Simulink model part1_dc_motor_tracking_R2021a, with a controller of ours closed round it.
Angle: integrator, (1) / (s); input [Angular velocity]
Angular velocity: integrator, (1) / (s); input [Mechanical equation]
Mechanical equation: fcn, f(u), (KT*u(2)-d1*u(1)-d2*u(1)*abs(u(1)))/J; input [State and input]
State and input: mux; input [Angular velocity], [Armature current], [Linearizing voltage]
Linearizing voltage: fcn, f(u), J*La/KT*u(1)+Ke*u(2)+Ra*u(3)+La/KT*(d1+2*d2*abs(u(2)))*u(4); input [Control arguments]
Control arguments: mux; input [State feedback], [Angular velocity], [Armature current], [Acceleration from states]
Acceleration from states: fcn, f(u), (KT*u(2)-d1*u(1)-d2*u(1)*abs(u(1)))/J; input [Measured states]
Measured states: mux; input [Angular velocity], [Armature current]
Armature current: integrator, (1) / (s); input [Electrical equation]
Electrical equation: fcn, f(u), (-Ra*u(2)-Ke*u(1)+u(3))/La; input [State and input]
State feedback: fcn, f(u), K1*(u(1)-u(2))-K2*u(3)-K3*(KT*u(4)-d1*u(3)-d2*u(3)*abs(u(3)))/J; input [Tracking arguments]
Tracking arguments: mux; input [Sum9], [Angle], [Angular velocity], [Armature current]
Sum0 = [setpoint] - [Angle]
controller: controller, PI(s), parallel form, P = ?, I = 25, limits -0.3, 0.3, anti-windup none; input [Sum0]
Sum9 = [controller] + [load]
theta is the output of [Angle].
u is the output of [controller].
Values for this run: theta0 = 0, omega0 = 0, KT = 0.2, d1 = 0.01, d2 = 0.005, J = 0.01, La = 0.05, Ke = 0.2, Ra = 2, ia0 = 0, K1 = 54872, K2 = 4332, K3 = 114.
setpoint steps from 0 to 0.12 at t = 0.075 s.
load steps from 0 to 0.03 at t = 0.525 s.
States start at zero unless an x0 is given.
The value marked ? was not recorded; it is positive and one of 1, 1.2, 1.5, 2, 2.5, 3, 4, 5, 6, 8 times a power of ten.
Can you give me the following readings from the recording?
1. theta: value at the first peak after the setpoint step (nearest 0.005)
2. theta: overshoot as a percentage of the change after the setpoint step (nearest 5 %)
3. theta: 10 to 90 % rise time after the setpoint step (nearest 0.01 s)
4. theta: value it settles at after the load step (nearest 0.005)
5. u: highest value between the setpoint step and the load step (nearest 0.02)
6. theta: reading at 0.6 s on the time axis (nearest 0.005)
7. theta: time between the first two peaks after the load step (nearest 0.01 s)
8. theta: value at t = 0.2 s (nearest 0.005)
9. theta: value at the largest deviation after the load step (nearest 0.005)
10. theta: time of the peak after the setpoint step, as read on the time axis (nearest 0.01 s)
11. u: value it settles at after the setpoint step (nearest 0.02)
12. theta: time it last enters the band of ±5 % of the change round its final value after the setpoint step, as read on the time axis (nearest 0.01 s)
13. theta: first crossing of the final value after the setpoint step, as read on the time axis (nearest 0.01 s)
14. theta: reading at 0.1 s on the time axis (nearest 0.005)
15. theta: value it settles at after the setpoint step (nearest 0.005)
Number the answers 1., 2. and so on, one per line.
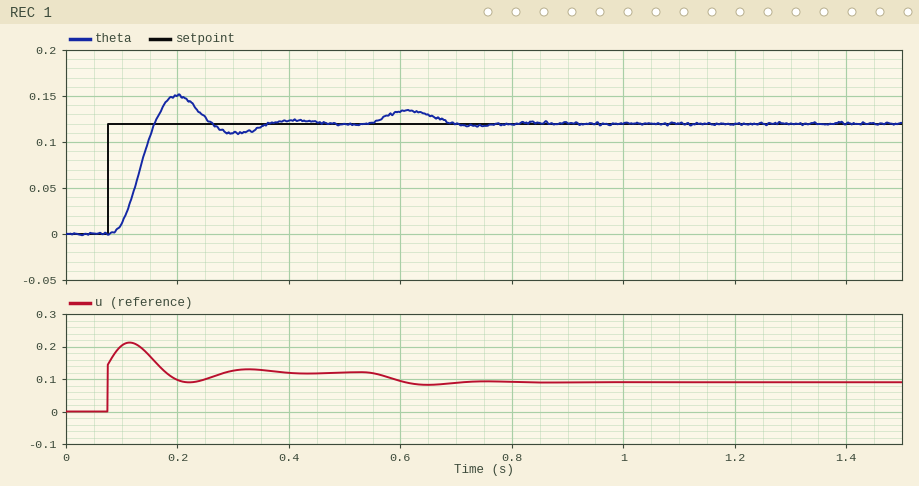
1. 0.150
2. 25 %
3. 0.05 s
4. 0.120
5. 0.22
6. 0.135
7. 0.22 s
8. 0.150
9. 0.135
10. 0.20 s
11. 0.12
12. 0.34 s
13. 0.16 s
14. 0.010
15. 0.120
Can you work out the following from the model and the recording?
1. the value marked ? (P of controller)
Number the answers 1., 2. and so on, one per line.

1. 1.2
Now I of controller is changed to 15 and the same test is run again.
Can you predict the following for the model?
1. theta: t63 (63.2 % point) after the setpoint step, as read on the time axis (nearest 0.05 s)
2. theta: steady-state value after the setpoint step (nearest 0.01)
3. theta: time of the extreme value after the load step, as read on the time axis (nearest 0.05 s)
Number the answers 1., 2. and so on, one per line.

1. 0.15 s
2. 0.12
3. 0.60 s
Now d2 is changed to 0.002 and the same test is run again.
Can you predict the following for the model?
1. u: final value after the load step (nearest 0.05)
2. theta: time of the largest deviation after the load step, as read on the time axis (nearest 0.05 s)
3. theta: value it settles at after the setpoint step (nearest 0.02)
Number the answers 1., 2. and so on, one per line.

1. 0.10
2. 0.60 s
3. 0.12
